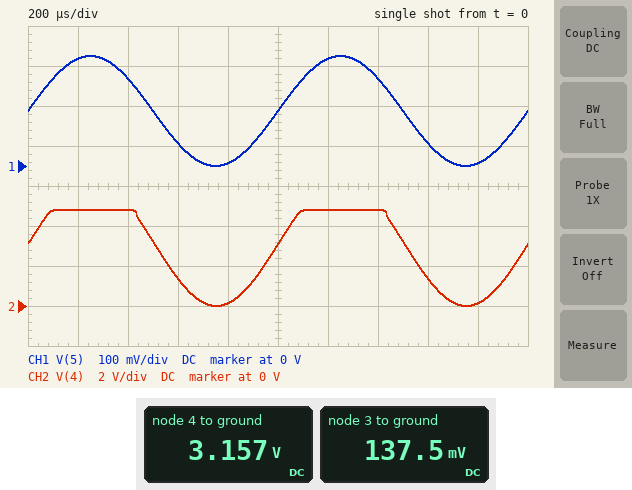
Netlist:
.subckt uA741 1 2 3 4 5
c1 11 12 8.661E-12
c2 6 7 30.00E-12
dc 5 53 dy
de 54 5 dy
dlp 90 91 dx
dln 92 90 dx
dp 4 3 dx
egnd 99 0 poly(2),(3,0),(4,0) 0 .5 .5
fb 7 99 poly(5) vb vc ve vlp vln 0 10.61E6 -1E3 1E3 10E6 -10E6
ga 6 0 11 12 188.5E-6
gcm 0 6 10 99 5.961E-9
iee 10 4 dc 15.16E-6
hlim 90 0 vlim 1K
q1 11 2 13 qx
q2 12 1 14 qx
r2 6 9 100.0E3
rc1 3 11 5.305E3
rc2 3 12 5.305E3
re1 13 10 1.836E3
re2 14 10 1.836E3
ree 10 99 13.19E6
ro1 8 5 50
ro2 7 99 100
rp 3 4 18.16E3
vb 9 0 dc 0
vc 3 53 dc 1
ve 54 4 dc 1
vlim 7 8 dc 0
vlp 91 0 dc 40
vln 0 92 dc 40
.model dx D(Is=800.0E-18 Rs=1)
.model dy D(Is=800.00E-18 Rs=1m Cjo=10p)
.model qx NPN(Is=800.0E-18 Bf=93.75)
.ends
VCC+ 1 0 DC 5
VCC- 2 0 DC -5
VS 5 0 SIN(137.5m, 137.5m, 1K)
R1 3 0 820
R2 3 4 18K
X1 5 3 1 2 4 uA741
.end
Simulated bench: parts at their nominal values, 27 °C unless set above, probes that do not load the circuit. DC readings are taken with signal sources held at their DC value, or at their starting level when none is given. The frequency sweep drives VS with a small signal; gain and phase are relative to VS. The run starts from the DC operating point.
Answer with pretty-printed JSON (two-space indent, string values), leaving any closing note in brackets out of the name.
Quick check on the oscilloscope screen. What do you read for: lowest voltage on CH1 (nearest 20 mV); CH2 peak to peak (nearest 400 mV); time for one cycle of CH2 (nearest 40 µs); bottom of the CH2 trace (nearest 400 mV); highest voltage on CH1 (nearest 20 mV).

{
  "lowest voltage on CH1": "0 V",
  "CH2 peak to peak": "4.8 V",
  "time for one cycle of CH2": "1.00 ms",
  "bottom of the CH2 trace": "0 V",
  "highest voltage on CH1": "280 mV"
}
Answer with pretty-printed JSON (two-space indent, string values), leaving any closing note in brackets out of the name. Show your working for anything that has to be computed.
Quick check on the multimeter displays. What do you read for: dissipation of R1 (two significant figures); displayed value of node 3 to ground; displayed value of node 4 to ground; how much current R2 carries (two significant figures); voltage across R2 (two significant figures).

{
  "dissipation of R1": "(137.5 mV)^2 / 820 Ω = 23 µW",
  "displayed value of node 3 to ground": "137.5 mV",
  "displayed value of node 4 to ground": "3.157 V",
  "how much current R2 carries": "(3.157 V - 137.5 mV) / 18 kΩ = 170 µA",
  "voltage across R2": "3.157 V - 137.5 mV = 3.0 V"
}
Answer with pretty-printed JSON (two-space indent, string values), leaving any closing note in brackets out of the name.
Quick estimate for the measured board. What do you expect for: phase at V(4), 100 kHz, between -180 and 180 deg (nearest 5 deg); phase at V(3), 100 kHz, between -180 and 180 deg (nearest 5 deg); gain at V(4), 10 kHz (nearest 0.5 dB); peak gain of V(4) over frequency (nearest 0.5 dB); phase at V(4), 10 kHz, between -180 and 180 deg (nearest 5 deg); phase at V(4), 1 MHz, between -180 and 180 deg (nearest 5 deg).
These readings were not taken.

{
  "phase at V(4), 100 kHz, between -180 and 180 deg": "-70 deg",
  "phase at V(3), 100 kHz, between -180 and 180 deg": "-70 deg",
  "gain at V(4), 10 kHz": "27.0 dB",
  "peak gain of V(4) over frequency": "27.0 dB",
  "phase at V(4), 10 kHz, between -180 and 180 deg": "-15 deg",
  "phase at V(4), 1 MHz, between -180 and 180 deg": "-120 deg"
}
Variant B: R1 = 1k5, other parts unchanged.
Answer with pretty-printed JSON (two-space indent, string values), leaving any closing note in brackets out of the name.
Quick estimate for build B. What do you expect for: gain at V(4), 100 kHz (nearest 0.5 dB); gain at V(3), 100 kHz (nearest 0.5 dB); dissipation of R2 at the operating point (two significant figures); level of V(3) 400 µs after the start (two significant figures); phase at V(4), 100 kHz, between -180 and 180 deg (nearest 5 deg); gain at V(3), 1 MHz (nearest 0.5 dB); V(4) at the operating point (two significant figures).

{
  "gain at V(4), 100 kHz": "18.0 dB",
  "gain at V(3), 100 kHz": "-4.0 dB",
  "dissipation of R2 at the operating point": "150 µW",
  "level of V(3) 400 µs after the start": "220 mV",
  "phase at V(4), 100 kHz, between -180 and 180 deg": "-55 deg",
  "gain at V(3), 1 MHz": "-23.5 dB",
  "V(4) at the operating point": "1.8 V"
}
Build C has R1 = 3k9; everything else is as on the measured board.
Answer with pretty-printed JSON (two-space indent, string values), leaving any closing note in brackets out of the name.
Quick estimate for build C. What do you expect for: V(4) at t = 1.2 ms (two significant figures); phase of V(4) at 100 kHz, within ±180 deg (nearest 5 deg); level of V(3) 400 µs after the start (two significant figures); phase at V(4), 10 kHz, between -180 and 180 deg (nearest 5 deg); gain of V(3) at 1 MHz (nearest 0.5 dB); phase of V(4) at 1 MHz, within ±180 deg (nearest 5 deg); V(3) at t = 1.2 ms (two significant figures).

{
  "V(4) at t = 1.2 ms": "1.5 V",
  "phase of V(4) at 100 kHz, within ±180 deg": "-30 deg",
  "level of V(3) 400 µs after the start": "220 mV",
  "phase at V(4), 10 kHz, between -180 and 180 deg": "-5 deg",
  "gain of V(3) at 1 MHz": "-16.0 dB",
  "phase of V(4) at 1 MHz, within ±180 deg": "-110 deg",
  "V(3) at t = 1.2 ms": "270 mV"
}
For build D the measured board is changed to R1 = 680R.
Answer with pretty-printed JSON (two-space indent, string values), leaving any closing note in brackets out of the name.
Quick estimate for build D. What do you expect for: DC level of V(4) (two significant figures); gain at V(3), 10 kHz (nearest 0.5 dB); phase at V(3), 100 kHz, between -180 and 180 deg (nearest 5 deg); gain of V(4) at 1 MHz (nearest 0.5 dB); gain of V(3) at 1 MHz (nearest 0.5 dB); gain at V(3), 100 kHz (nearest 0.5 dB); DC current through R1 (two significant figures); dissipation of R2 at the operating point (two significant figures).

{
  "DC level of V(4)": "3.8 V",
  "gain at V(3), 10 kHz": "-0.5 dB",
  "phase at V(3), 100 kHz, between -180 and 180 deg": "-75 deg",
  "gain of V(4) at 1 MHz": "-1.0 dB",
  "gain of V(3) at 1 MHz": "-30.0 dB",
  "gain at V(3), 100 kHz": "-9.0 dB",
  "DC current through R1": "200 µA",
  "dissipation of R2 at the operating point": "740 µW"
}
